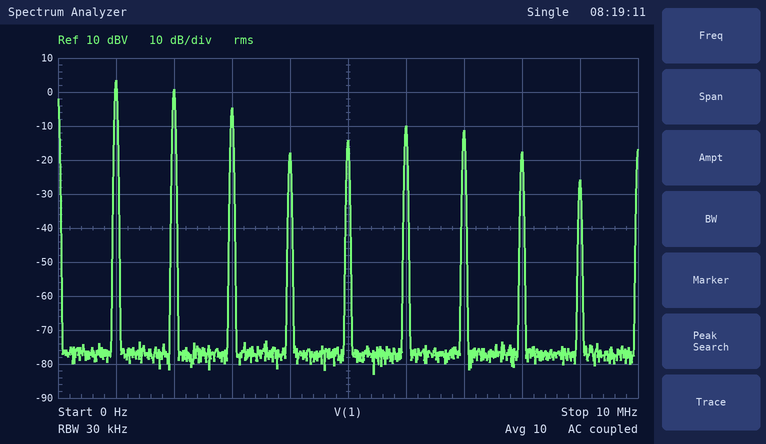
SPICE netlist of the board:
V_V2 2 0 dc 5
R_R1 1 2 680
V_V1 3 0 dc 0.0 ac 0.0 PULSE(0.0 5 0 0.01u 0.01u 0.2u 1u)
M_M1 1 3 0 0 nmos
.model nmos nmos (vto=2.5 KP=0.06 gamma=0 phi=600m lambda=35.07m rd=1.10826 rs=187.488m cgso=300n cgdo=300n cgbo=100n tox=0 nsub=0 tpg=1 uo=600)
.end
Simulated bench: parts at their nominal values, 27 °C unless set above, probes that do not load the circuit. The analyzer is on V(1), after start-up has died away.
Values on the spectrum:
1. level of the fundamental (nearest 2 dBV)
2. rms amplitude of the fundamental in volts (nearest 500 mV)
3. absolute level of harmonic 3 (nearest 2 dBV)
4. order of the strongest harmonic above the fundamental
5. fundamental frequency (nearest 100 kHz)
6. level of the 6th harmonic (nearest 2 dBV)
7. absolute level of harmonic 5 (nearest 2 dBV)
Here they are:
4 dBV
1.5 V
-4 dBV
2
1.0 MHz
-10 dBV
-14 dBV
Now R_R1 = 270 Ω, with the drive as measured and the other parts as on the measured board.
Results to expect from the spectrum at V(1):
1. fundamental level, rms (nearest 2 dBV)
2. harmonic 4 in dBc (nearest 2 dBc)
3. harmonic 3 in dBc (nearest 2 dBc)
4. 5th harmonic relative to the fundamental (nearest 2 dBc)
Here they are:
2 dBV
-16 dBc
-6 dBc
-22 dBc
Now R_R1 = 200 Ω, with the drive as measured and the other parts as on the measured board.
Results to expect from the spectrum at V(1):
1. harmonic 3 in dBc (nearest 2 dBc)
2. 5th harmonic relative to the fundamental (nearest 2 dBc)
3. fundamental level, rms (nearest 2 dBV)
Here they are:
-6 dBc
-24 dBc
2 dBV
